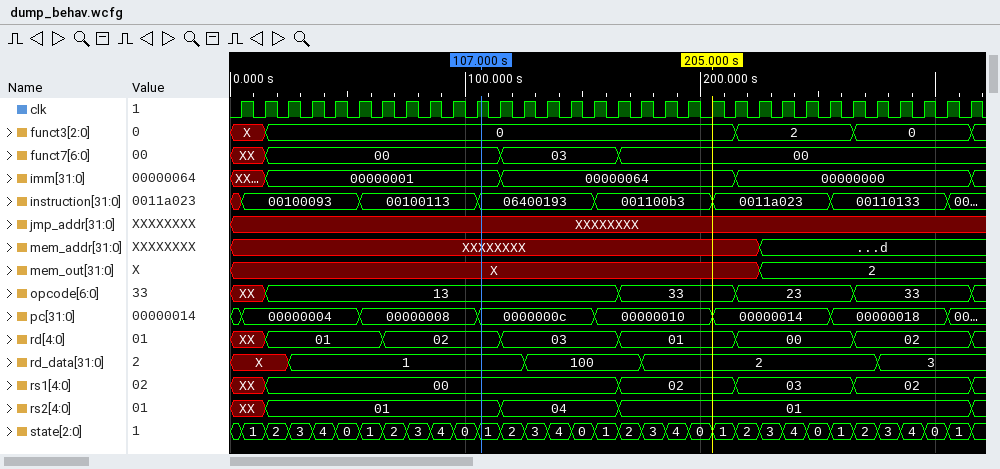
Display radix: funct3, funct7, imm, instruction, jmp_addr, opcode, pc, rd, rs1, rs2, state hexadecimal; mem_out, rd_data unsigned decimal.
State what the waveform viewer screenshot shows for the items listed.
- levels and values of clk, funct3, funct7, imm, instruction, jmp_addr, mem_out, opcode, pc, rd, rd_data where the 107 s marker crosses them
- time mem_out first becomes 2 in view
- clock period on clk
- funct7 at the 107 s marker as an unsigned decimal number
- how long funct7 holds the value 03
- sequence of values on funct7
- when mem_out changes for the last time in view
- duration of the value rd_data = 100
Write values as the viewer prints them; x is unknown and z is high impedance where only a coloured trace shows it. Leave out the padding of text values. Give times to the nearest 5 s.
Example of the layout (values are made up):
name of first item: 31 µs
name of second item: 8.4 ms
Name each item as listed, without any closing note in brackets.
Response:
levels and values of clk, funct3, funct7, imm, instruction, jmp_addr, mem_out, opcode, pc, rd, rd_data where the 107 s marker crosses them: clk=1, funct3=0, funct7=00, imm=00000001, instruction=06400193, jmp_addr=XXXXXXXX, mem_out=X, opcode=13, pc=0000000c, rd=02, rd_data=1
time mem_out first becomes 2 in view: 225 s
clock period on clk: 10 s
funct7 at the 107 s marker as an unsigned decimal number: 0
how long funct7 holds the value 03: 50 s
sequence of values on funct7: XX, 00, 03, 00
when mem_out changes for the last time in view: 225 s
duration of the value rd_data = 100: 50 s
